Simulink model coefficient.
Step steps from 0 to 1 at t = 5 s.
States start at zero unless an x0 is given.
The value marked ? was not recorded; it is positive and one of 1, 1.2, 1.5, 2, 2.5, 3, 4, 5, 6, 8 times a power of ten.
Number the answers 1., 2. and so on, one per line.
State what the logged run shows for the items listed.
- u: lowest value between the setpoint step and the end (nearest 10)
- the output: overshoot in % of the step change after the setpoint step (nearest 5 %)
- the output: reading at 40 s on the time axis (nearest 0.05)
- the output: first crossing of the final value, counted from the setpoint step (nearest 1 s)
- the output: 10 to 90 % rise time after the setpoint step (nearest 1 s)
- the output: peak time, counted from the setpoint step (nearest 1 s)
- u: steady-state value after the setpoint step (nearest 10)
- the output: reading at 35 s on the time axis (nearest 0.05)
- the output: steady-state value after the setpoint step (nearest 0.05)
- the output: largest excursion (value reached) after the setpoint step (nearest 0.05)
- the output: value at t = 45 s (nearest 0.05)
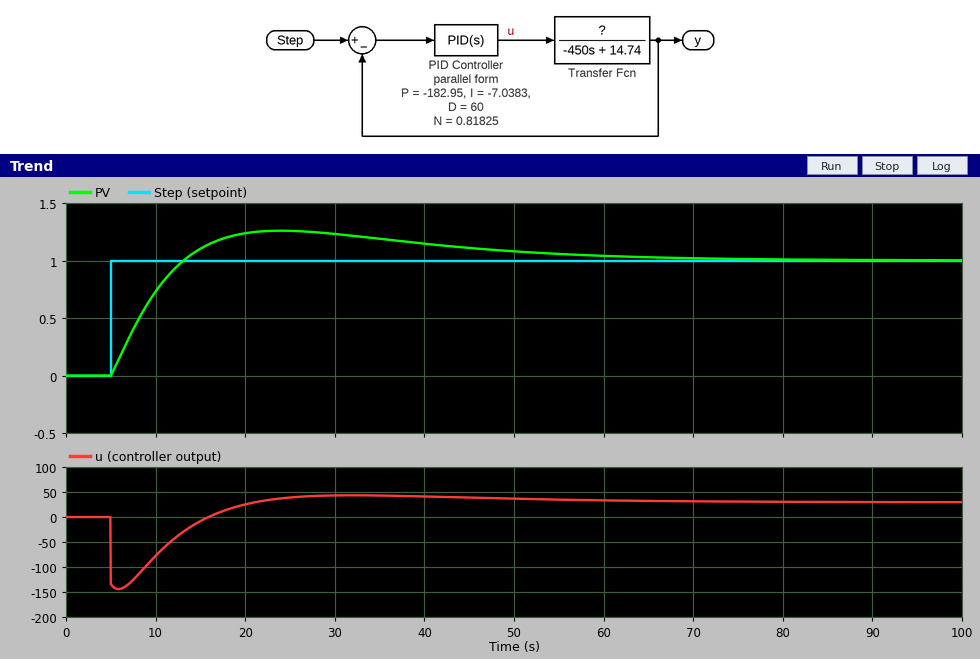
1. -140
2. 25 %
3. 1.15
4. 8 s
5. 6 s
6. 19 s
7. 30
8. 1.20
9. 1.00
10. 1.25
11. 1.10
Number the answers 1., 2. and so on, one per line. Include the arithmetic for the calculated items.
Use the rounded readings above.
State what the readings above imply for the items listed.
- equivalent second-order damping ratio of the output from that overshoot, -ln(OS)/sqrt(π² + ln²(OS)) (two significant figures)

1. ln(0.25) = -1.386; 1.386 / sqrt(9.870 + 1.922) = 0.40
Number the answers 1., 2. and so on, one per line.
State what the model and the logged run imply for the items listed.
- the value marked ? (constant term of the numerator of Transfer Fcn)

1. 0.5
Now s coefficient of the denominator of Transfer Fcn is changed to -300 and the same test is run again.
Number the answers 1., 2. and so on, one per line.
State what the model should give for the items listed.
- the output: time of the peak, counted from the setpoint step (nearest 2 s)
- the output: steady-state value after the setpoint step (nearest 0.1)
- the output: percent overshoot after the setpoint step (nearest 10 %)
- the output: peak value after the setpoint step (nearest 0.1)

1. 14 s
2. 1.0
3. 20 %
4. 1.2
